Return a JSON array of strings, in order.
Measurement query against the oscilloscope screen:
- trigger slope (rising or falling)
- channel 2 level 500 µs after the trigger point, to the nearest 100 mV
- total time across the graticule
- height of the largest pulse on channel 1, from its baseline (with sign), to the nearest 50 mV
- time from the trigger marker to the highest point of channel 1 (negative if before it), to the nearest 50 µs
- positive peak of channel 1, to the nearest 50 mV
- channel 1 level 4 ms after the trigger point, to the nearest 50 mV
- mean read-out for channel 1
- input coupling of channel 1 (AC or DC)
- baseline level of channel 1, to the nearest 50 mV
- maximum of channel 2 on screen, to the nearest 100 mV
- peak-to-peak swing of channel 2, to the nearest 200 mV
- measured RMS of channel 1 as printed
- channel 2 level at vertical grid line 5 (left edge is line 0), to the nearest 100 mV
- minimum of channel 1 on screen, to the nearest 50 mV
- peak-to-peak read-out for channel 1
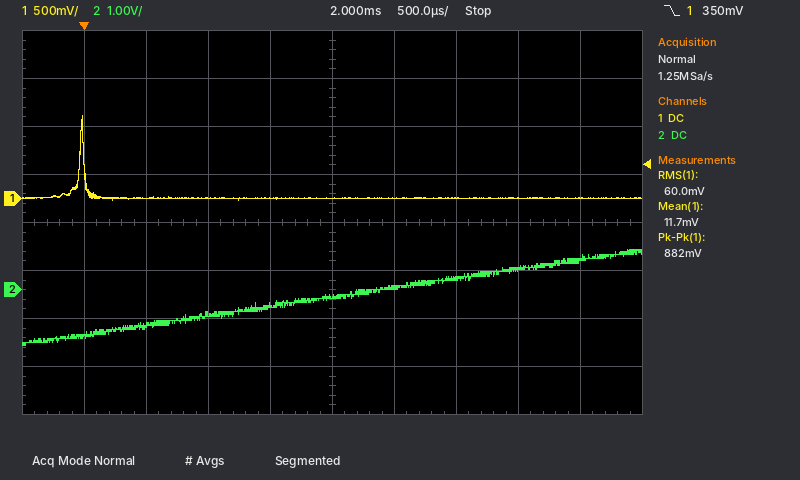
["falling", "-800 mV", "5 ms", "+850 mV", "0 µs", "850 mV", "0 mV", "11.7 mV", "DC", "0 mV", "800 mV", "2.0 V", "60.0 mV", "-100 mV", "0 mV", "882 mV"]
